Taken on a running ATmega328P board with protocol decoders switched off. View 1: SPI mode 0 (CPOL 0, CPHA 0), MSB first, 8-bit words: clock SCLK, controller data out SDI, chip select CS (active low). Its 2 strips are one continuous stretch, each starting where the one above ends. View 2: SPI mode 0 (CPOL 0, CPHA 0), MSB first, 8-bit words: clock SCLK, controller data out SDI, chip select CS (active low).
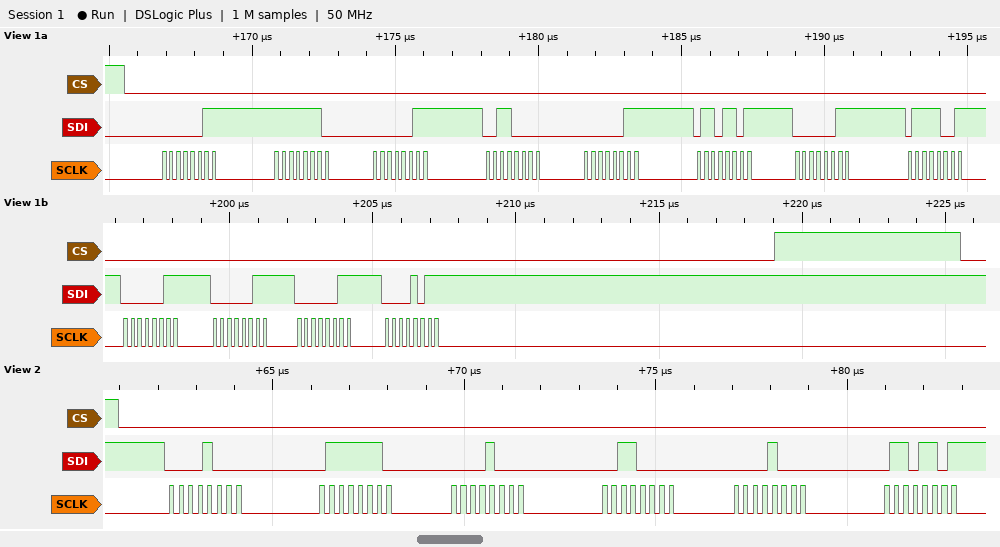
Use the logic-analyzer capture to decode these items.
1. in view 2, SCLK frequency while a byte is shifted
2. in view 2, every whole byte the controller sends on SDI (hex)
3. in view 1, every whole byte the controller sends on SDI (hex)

4 MHz
0x08 0x7E 0x08 0x30 0x08 0x6D
03 FE 03 30 03 6D 03 79 03 03 03 0B
